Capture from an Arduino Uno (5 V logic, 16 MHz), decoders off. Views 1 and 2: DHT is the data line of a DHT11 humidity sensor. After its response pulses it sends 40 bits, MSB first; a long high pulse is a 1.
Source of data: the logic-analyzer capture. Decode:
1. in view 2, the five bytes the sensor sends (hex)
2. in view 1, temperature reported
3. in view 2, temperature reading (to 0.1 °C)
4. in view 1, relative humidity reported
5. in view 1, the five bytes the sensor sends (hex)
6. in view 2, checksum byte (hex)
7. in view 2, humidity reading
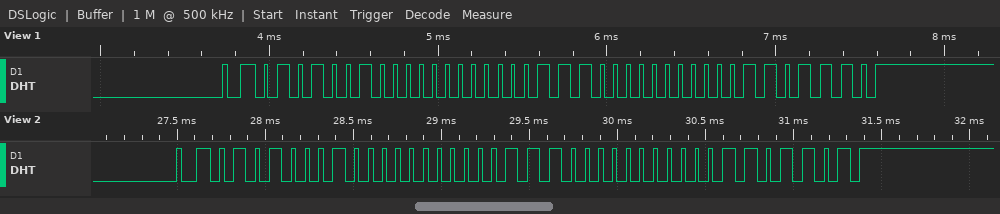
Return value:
51 00 1C 00 6D
28.0 °C
28.0 °C
82 %
52 00 1C 00 6E
0x6D
81 %
